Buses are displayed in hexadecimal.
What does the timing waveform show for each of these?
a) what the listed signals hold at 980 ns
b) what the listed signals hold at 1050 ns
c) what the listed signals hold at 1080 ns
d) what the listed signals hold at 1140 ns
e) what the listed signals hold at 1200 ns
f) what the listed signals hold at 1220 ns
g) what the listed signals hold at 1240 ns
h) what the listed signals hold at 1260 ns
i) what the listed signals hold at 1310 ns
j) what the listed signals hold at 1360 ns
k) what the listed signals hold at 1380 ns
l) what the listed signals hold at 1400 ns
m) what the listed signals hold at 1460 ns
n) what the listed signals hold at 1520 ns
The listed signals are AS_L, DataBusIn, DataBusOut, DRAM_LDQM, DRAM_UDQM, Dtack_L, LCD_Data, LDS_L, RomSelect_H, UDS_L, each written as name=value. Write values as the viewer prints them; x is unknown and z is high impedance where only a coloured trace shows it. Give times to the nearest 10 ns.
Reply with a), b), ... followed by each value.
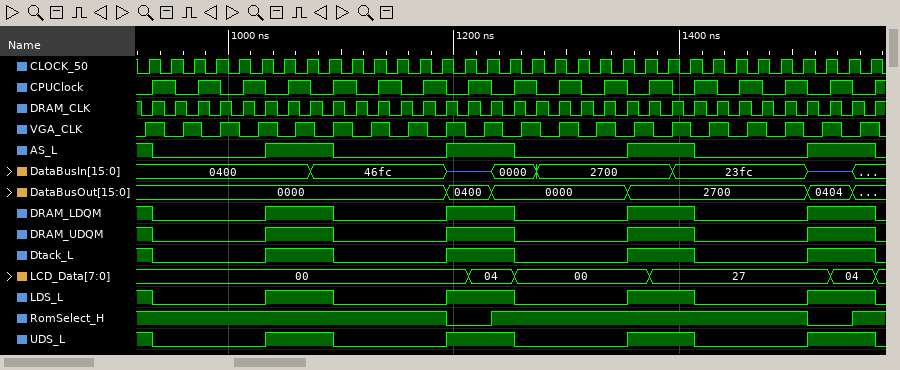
a) AS_L=0, DataBusIn=0400, DataBusOut=0000, DRAM_LDQM=0, DRAM_UDQM=0, Dtack_L=0, LCD_Data=00, LDS_L=0, RomSelect_H=1, UDS_L=0
b) AS_L=1, DataBusIn=0400, DataBusOut=0000, DRAM_LDQM=1, DRAM_UDQM=1, Dtack_L=1, LCD_Data=00, LDS_L=1, RomSelect_H=1, UDS_L=1
c) AS_L=1, DataBusIn=46fc, DataBusOut=0000, DRAM_LDQM=1, DRAM_UDQM=1, Dtack_L=1, LCD_Data=00, LDS_L=1, RomSelect_H=1, UDS_L=1
d) AS_L=0, DataBusIn=46fc, DataBusOut=0000, DRAM_LDQM=0, DRAM_UDQM=0, Dtack_L=0, LCD_Data=00, LDS_L=0, RomSelect_H=1, UDS_L=0
e) AS_L=1, DataBusIn=z, DataBusOut=0400, DRAM_LDQM=1, DRAM_UDQM=1, Dtack_L=1, LCD_Data=00, LDS_L=1, RomSelect_H=0, UDS_L=1
f) AS_L=1, DataBusIn=z, DataBusOut=0400, DRAM_LDQM=1, DRAM_UDQM=1, Dtack_L=1, LCD_Data=04, LDS_L=1, RomSelect_H=0, UDS_L=1
g) AS_L=1, DataBusIn=0000, DataBusOut=0000, DRAM_LDQM=1, DRAM_UDQM=1, Dtack_L=1, LCD_Data=04, LDS_L=1, RomSelect_H=1, UDS_L=1
h) AS_L=0, DataBusIn=0000, DataBusOut=0000, DRAM_LDQM=0, DRAM_UDQM=0, Dtack_L=0, LCD_Data=00, LDS_L=0, RomSelect_H=1, UDS_L=0
i) AS_L=0, DataBusIn=2700, DataBusOut=0000, DRAM_LDQM=0, DRAM_UDQM=0, Dtack_L=0, LCD_Data=00, LDS_L=0, RomSelect_H=1, UDS_L=0
j) AS_L=1, DataBusIn=2700, DataBusOut=2700, DRAM_LDQM=1, DRAM_UDQM=1, Dtack_L=1, LCD_Data=00, LDS_L=1, RomSelect_H=1, UDS_L=1
k) AS_L=1, DataBusIn=2700, DataBusOut=2700, DRAM_LDQM=1, DRAM_UDQM=1, Dtack_L=1, LCD_Data=27, LDS_L=1, RomSelect_H=1, UDS_L=1
l) AS_L=1, DataBusIn=23fc, DataBusOut=2700, DRAM_LDQM=1, DRAM_UDQM=1, Dtack_L=1, LCD_Data=27, LDS_L=1, RomSelect_H=1, UDS_L=1
m) AS_L=0, DataBusIn=23fc, DataBusOut=2700, DRAM_LDQM=0, DRAM_UDQM=0, Dtack_L=0, LCD_Data=27, LDS_L=0, RomSelect_H=1, UDS_L=0
n) AS_L=1, DataBusIn=z, DataBusOut=0404, DRAM_LDQM=1, DRAM_UDQM=1, Dtack_L=1, LCD_Data=27, LDS_L=1, RomSelect_H=0, UDS_L=1
